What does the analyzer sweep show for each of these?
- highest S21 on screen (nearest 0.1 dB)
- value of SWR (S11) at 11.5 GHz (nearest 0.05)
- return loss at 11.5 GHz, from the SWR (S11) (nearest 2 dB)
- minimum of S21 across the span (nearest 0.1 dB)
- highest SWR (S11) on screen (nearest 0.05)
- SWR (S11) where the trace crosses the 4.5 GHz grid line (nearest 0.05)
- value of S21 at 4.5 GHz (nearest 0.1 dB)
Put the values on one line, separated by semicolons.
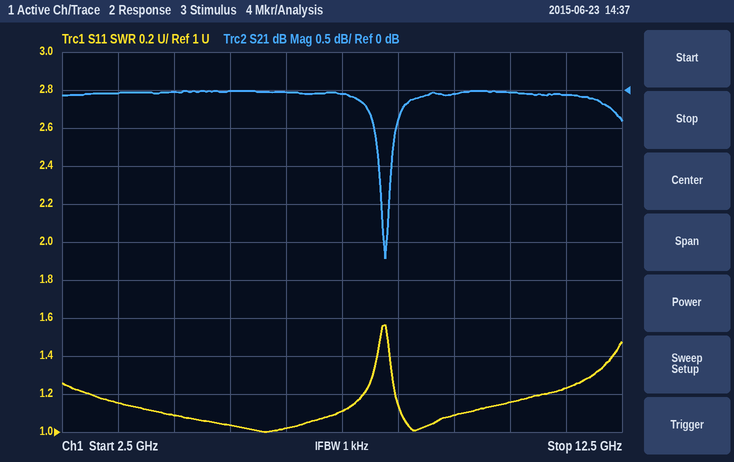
0.0 dB; 1.25; 20 dB; -2.2 dB; 1.55; 1.10; 0.0 dB
